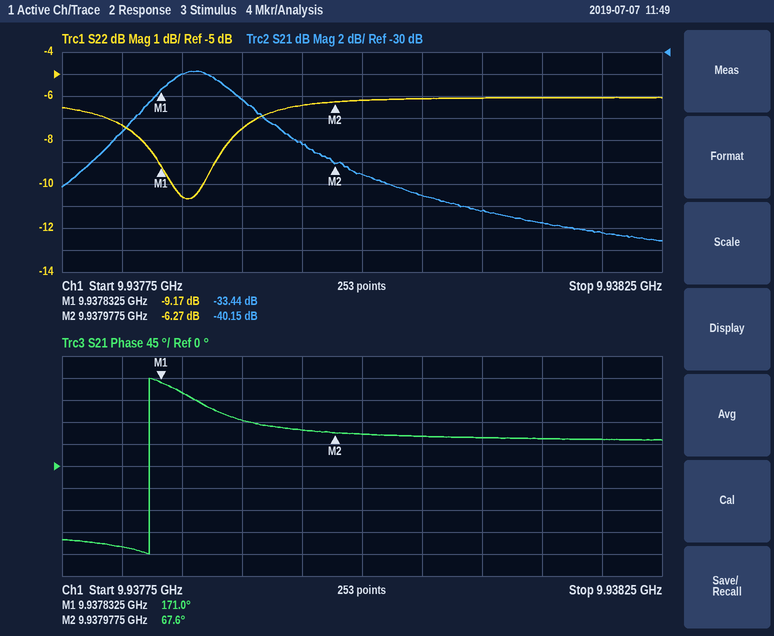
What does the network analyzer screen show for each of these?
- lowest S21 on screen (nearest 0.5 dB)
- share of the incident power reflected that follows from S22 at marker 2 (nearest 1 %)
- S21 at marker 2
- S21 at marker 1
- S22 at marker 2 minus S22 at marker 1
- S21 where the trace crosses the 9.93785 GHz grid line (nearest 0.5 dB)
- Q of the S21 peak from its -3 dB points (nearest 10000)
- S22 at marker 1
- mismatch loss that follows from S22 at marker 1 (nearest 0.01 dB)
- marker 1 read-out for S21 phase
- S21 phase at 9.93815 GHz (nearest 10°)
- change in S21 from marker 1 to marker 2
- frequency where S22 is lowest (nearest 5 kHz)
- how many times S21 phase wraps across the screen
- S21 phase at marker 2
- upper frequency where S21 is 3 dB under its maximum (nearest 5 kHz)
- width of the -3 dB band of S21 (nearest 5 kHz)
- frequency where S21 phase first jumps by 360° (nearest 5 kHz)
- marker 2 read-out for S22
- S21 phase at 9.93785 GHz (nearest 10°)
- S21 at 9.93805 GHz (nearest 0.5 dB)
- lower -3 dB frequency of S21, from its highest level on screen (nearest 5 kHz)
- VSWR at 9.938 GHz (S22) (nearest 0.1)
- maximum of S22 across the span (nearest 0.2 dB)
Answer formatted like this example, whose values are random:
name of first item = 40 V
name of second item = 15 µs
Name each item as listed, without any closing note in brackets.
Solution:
lowest S21 on screen = -47.0 dB
share of the incident power reflected that follows from S22 at marker 2 = 24 %
S21 at marker 2 = -40.15 dB
S21 at marker 1 = -33.44 dB
S22 at marker 2 minus S22 at marker 1 = 2.90 dB
S21 where the trace crosses the 9.93785 GHz grid line = -32.0 dB
Q of the S21 peak from its -3 dB points = 120000
S22 at marker 1 = -9.17 dB
mismatch loss that follows from S22 at marker 1 = 0.56 dB
marker 1 read-out for S21 phase = 171.0°
S21 phase at 9.93815 GHz = 60°
change in S21 from marker 1 to marker 2 = -6.71 dB
frequency where S22 is lowest = 9.937855 GHz
how many times S21 phase wraps across the screen = 1
S21 phase at marker 2 = 67.6°
upper frequency where S21 is 3 dB under its maximum = 9.937905 GHz
width of the -3 dB band of S21 = 85 kHz
frequency where S21 phase first jumps by 360° = 9.937825 GHz
marker 2 read-out for S22 = -6.27 dB
S21 phase at 9.93785 GHz = 150°
S21 at 9.93805 GHz = -43.0 dB
lower -3 dB frequency of S21, from its highest level on screen = 9.937820 GHz
VSWR at 9.938 GHz (S22) = 2.9
maximum of S22 across the span = -6.0 dB
